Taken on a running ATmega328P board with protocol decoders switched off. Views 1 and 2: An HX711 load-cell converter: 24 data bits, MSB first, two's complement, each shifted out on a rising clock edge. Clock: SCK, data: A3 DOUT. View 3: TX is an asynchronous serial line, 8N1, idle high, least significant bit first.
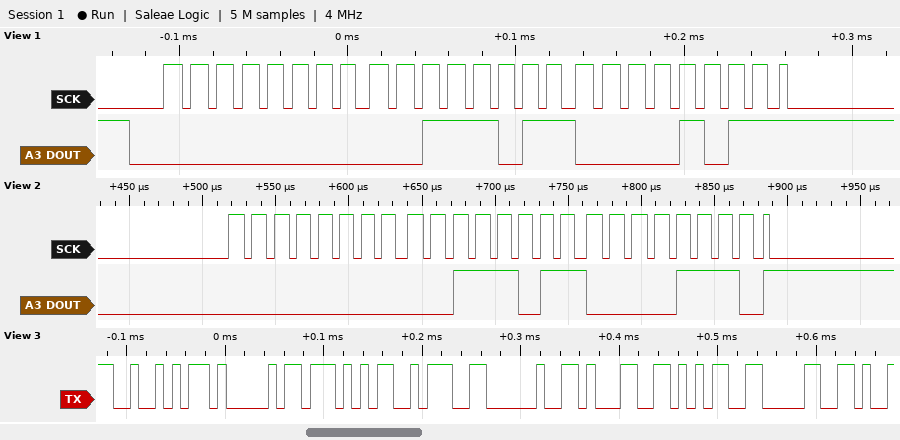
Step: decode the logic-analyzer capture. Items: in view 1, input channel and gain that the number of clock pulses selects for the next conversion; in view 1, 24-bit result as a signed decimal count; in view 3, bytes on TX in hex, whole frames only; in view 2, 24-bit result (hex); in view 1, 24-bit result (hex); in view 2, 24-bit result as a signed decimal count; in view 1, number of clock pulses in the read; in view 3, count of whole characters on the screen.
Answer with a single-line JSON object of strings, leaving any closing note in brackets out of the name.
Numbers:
{"in view 1, input channel and gain that the number of clock pulses selects for the next conversion": "channel A, gain 128", "in view 1, 24-bit result as a signed decimal count": "15115", "in view 3, bytes on TX in hex, whole frames only": "52 41 57 3A 20 31 35 30", "in view 2, 24-bit result": "0x003B0E", "in view 1, 24-bit result": "0x003B0B", "in view 2, 24-bit result as a signed decimal count": "15118", "in view 1, number of clock pulses in the read": "25", "in view 3, count of whole characters on the screen": "8"}
